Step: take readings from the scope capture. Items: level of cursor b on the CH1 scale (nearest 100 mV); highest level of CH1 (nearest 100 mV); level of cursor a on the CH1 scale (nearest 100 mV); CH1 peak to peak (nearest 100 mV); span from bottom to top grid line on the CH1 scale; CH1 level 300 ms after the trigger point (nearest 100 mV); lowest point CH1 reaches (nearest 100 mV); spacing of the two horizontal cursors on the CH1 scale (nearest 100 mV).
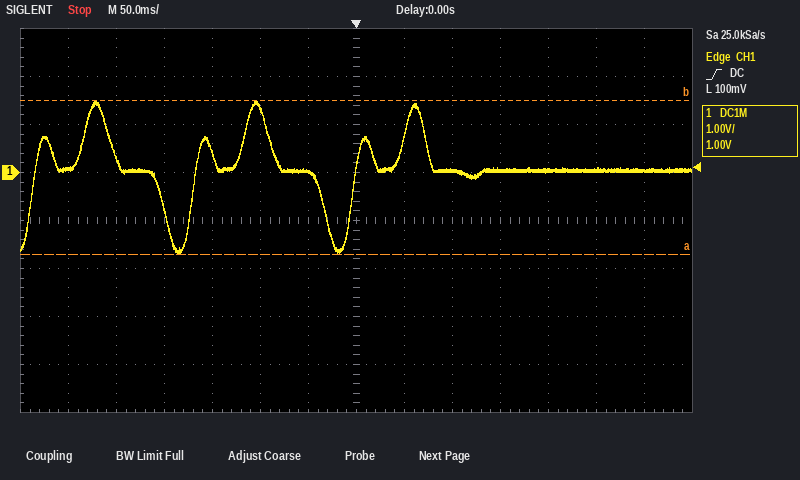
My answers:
1.5 V
1.5 V
-1.7 V
3.2 V
8 V
0.0 V
-1.7 V
3.2 V
